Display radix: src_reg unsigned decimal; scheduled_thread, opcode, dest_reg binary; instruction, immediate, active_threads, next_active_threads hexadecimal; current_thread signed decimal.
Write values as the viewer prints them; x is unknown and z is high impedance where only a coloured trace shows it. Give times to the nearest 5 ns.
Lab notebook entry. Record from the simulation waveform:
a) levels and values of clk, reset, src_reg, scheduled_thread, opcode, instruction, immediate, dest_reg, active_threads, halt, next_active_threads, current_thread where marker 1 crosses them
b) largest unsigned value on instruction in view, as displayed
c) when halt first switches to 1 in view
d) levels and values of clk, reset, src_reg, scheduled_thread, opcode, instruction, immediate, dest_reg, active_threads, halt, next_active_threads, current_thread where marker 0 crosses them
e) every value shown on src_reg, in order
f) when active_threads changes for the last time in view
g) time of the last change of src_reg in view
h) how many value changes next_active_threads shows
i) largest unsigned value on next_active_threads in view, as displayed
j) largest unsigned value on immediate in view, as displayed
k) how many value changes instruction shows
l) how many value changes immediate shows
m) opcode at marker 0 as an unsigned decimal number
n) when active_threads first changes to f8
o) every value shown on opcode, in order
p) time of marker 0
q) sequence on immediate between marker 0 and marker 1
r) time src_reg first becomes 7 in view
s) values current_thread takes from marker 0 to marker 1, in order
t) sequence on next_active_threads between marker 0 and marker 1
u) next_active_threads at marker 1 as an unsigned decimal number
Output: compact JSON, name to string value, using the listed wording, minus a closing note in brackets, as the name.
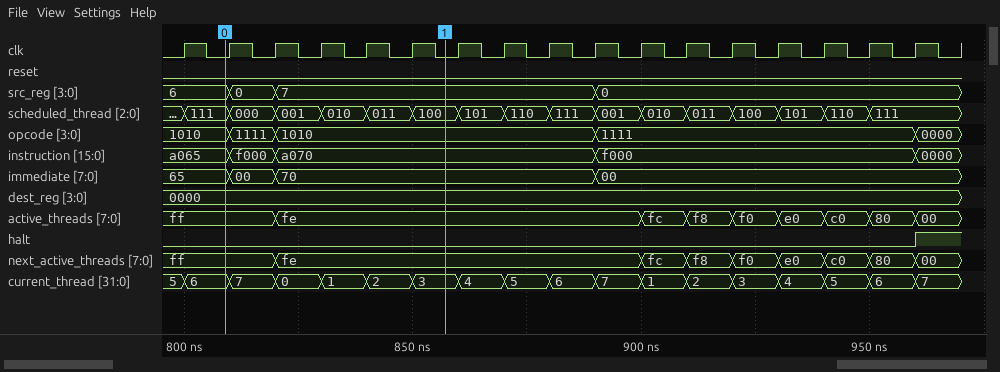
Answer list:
{"levels and values of clk, reset, src_reg, scheduled_thread, opcode, instruction, immediate, dest_reg, active_threads, halt, next_active_threads, current_thread where marker 1 crosses them": "clk=0, reset=0, src_reg=7, scheduled_thread=100, opcode=1010, instruction=a070, immediate=70, dest_reg=0000, active_threads=fe, halt=0, next_active_threads=fe, current_thread=3", "largest unsigned value on instruction in view, as displayed": "f000", "when halt first switches to 1 in view": "960 ns", "levels and values of clk, reset, src_reg, scheduled_thread, opcode, instruction, immediate, dest_reg, active_threads, halt, next_active_threads, current_thread where marker 0 crosses them": "clk=0, reset=0, src_reg=6, scheduled_thread=111, opcode=1010, instruction=a065, immediate=65, dest_reg=0000, active_threads=ff, halt=0, next_active_threads=ff, current_thread=6", "every value shown on src_reg, in order": "6, 0, 7, 0", "when active_threads changes for the last time in view": "960 ns", "time of the last change of src_reg in view": "890 ns", "how many value changes next_active_threads shows": "8", "largest unsigned value on next_active_threads in view, as displayed": "ff", "largest unsigned value on immediate in view, as displayed": "70", "how many value changes instruction shows": "4", "how many value changes immediate shows": "3", "opcode at marker 0 as an unsigned decimal number": "10", "when active_threads first changes to f8": "910 ns", "every value shown on opcode, in order": "1010, 1111, 1010, 1111, 0000", "time of marker 0": "810 ns", "sequence on immediate between marker 0 and marker 1": "65, 00, 70", "time src_reg first becomes 7 in view": "820 ns", "values current_thread takes from marker 0 to marker 1, in order": "6, 7, 0, 1, 2, 3", "sequence on next_active_threads between marker 0 and marker 1": "ff, fe", "next_active_threads at marker 1 as an unsigned decimal number": "254"}
